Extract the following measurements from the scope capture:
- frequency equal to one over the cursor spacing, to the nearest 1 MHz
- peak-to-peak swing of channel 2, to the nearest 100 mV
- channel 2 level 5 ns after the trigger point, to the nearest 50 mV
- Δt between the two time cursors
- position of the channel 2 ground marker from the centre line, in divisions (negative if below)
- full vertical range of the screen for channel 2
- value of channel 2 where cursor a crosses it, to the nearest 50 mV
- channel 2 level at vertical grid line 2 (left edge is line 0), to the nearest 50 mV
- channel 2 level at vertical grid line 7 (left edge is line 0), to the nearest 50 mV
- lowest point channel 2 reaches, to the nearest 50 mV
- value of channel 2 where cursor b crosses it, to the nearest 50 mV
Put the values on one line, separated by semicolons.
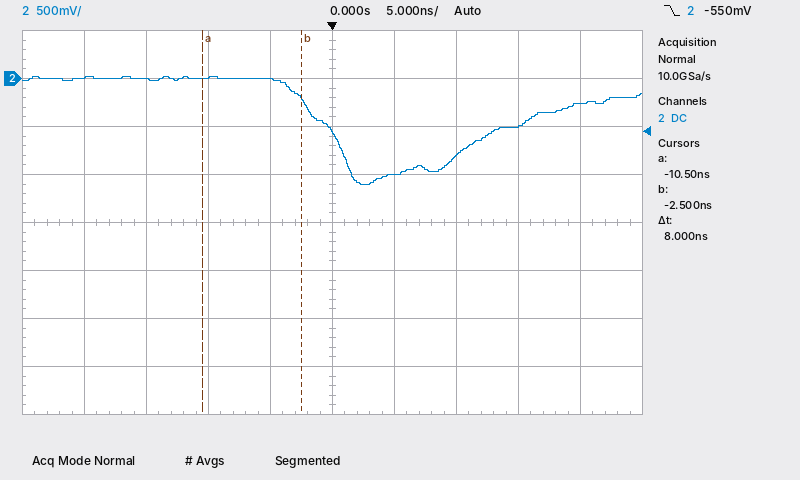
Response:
125 MHz; 1.10 V; -1.00 V; 8 ns; +3.0 div; 4 V; 0 mV; 0 mV; -800 mV; -1.10 V; -200 mV
